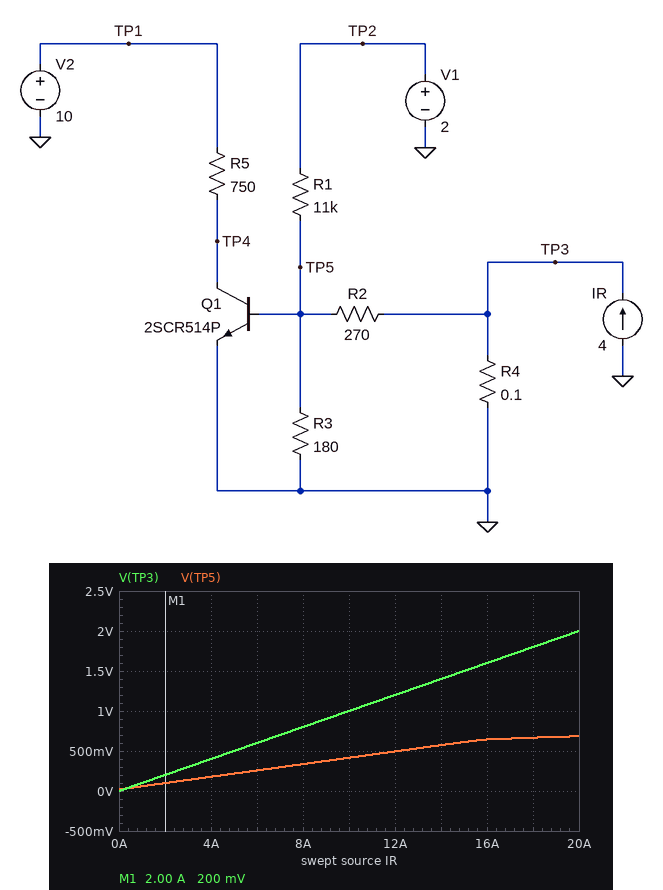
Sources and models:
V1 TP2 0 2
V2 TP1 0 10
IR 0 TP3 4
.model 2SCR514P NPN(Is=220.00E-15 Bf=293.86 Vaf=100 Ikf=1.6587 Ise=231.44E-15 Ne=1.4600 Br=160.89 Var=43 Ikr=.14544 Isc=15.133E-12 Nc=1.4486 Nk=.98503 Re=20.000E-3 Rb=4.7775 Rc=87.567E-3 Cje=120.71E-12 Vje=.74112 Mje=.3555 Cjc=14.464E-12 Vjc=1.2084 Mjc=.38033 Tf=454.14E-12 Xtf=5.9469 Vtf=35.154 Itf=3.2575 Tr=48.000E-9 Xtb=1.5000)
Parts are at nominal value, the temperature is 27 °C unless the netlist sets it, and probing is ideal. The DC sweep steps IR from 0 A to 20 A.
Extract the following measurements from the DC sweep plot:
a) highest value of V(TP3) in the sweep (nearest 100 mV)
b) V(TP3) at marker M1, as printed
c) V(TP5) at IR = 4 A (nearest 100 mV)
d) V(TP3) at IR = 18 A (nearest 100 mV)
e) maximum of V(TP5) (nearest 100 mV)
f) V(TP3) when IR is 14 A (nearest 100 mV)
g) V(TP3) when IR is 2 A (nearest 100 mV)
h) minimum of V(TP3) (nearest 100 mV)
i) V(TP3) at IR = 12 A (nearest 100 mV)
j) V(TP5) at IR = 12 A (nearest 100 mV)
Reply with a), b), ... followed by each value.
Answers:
a) 2.0 V
b) 200 mV
c) 200 mV
d) 1.8 V
e) 700 mV
f) 1.4 V
g) 200 mV
h) 0 V
i) 1.2 V
j) 500 mV
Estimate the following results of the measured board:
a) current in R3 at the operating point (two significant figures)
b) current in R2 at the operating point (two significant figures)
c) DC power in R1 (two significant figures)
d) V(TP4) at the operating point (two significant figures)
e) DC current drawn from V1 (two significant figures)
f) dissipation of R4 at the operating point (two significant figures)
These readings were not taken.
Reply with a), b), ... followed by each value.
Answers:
a) 990 µA
b) 820 µA
c) 300 µW
d) 10 V
e) 170 µA
f) 1.6 W
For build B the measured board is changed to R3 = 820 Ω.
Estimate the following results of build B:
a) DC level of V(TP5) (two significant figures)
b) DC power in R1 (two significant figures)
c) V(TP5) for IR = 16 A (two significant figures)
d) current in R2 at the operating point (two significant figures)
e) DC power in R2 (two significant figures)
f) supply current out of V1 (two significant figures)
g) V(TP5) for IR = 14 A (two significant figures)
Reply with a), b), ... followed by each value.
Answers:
a) 330 mV
b) 250 µW
c) 710 mV
d) 250 µA
e) 17 µW
f) 150 µA
g) 700 mV
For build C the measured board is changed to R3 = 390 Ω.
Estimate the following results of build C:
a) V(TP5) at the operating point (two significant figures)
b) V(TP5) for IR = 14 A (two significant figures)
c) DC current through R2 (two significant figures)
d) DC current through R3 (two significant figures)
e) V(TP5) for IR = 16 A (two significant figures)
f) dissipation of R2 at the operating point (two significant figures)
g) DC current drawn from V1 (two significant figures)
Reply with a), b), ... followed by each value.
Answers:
a) 260 mV
b) 680 mV
c) 510 µA
d) 670 µA
e) 700 mV
f) 71 µW
g) 160 µA
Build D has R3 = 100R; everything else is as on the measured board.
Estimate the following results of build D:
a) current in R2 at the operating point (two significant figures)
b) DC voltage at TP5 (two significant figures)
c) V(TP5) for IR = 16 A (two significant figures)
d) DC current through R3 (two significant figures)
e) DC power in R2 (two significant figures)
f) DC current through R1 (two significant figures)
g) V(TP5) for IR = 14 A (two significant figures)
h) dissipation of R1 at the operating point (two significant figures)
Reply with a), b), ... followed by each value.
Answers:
a) 1.0 mA
b) 120 mV
c) 440 mV
d) 1.2 mA
e) 290 µW
f) 170 µA
g) 390 mV
h) 320 µW
